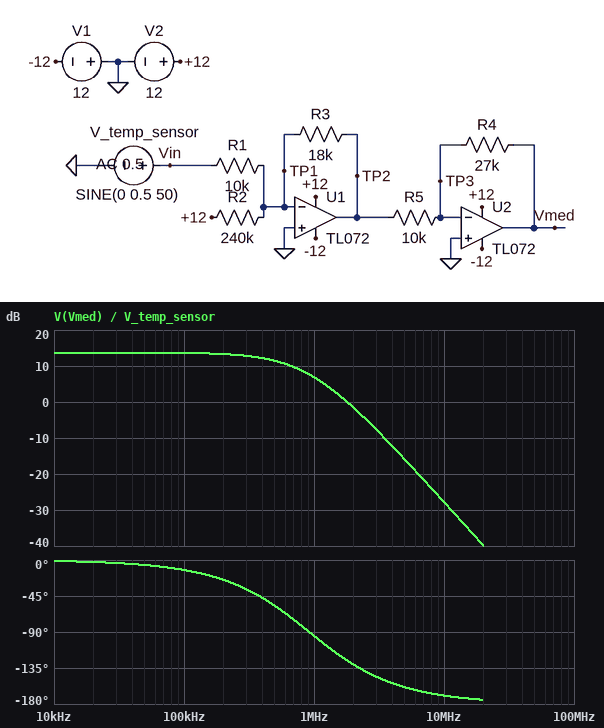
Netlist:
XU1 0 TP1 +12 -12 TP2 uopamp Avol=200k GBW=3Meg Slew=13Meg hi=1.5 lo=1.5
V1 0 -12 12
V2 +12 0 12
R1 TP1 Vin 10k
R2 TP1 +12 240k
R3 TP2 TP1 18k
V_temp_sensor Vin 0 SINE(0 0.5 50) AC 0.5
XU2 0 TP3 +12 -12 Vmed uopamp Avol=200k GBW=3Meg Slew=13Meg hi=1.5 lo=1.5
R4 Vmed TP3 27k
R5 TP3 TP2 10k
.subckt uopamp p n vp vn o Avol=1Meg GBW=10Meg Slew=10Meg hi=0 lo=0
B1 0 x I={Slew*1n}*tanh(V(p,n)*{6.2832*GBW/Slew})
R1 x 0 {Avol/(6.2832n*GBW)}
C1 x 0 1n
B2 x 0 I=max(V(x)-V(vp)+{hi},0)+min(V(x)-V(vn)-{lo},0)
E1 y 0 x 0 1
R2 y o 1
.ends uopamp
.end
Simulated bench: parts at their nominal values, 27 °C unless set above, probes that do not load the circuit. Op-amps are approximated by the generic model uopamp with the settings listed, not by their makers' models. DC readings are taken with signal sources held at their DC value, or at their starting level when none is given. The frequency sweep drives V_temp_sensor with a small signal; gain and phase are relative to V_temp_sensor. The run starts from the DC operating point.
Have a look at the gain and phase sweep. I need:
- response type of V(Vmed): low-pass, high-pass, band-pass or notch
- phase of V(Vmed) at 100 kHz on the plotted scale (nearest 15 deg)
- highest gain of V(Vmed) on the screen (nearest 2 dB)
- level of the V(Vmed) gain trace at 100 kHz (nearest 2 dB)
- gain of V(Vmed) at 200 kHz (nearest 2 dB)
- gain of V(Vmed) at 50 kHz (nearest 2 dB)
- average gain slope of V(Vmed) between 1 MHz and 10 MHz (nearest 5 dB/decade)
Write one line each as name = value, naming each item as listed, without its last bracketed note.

response type of V(Vmed): low-pass, high-pass, band-pass or notch = low-pass
phase of V(Vmed) at 100 kHz on the plotted scale = -15 deg
highest gain of V(Vmed) on the screen = 14 dB
level of the V(Vmed) gain trace at 100 kHz = 14 dB
gain of V(Vmed) at 200 kHz = 14 dB
gain of V(Vmed) at 50 kHz = 14 dB
average gain slope of V(Vmed) between 1 MHz and 10 MHz = -35 dB/decade
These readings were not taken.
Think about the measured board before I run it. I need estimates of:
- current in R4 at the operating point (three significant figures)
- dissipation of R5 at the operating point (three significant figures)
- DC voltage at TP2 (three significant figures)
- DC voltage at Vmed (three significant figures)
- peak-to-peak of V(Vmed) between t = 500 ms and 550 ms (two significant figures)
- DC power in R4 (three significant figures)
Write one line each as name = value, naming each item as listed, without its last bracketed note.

current in R4 at the operating point = 90.0 µA
dissipation of R5 at the operating point = 81.0 µW
DC voltage at TP2 = -900 mV
DC voltage at Vmed = 2.43 V
peak-to-peak of V(Vmed) between t = 500 ms and 550 ms = 4.9 V
DC power in R4 = 219 µW
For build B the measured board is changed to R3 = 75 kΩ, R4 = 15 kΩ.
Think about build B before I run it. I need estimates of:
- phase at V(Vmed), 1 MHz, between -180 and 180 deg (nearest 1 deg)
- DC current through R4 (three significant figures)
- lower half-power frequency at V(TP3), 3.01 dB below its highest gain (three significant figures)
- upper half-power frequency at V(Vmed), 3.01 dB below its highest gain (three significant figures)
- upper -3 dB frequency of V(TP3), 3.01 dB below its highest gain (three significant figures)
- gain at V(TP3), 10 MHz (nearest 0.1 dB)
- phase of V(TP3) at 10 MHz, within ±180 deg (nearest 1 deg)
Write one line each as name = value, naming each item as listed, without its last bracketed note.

phase at V(Vmed), 1 MHz, between -180 and 180 deg = -111 deg
DC current through R4 = 375 µA
lower half-power frequency at V(TP3), 3.01 dB below its highest gain = 231 kHz
upper half-power frequency at V(Vmed), 3.01 dB below its highest gain = 317 kHz
upper -3 dB frequency of V(TP3), 3.01 dB below its highest gain = 1.77 MHz
gain at V(TP3), 10 MHz = -16.4 dB
phase of V(TP3) at 10 MHz, within ±180 deg = 99 deg
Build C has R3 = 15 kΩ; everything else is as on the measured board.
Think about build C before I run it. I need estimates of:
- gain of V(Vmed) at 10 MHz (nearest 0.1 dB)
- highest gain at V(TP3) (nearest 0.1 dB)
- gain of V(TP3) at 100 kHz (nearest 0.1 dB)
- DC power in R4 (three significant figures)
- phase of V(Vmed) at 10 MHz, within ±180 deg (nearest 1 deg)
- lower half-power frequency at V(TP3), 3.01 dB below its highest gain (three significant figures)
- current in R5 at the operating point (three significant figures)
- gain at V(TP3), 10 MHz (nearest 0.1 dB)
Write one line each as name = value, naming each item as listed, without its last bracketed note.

gain of V(Vmed) at 10 MHz = -28.4 dB
highest gain at V(TP3) = -3.8 dB
gain of V(TP3) at 100 kHz = -17.5 dB
DC power in R4 = 152 µW
phase of V(Vmed) at 10 MHz, within ±180 deg = -169 deg
lower half-power frequency at V(TP3), 3.01 dB below its highest gain = 399 kHz
current in R5 at the operating point = 75.0 µA
gain at V(TP3), 10 MHz = -17.9 dB
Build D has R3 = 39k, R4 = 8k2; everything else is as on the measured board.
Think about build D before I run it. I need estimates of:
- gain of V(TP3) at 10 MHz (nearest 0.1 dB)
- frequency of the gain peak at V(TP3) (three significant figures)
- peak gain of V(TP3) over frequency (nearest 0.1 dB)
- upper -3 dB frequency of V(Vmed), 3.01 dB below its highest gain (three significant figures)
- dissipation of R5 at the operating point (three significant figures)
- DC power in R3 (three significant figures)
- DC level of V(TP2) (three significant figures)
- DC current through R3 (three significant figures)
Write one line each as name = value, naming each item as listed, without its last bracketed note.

gain of V(TP3) at 10 MHz = -19.8 dB
frequency of the gain peak at V(TP3) = 988 kHz
peak gain of V(TP3) over frequency = -6.7 dB
upper -3 dB frequency of V(Vmed), 3.01 dB below its highest gain = 533 kHz
dissipation of R5 at the operating point = 380 µW
DC power in R3 = 97.5 µW
DC level of V(TP2) = -1.95 V
DC current through R3 = 50.0 µA
